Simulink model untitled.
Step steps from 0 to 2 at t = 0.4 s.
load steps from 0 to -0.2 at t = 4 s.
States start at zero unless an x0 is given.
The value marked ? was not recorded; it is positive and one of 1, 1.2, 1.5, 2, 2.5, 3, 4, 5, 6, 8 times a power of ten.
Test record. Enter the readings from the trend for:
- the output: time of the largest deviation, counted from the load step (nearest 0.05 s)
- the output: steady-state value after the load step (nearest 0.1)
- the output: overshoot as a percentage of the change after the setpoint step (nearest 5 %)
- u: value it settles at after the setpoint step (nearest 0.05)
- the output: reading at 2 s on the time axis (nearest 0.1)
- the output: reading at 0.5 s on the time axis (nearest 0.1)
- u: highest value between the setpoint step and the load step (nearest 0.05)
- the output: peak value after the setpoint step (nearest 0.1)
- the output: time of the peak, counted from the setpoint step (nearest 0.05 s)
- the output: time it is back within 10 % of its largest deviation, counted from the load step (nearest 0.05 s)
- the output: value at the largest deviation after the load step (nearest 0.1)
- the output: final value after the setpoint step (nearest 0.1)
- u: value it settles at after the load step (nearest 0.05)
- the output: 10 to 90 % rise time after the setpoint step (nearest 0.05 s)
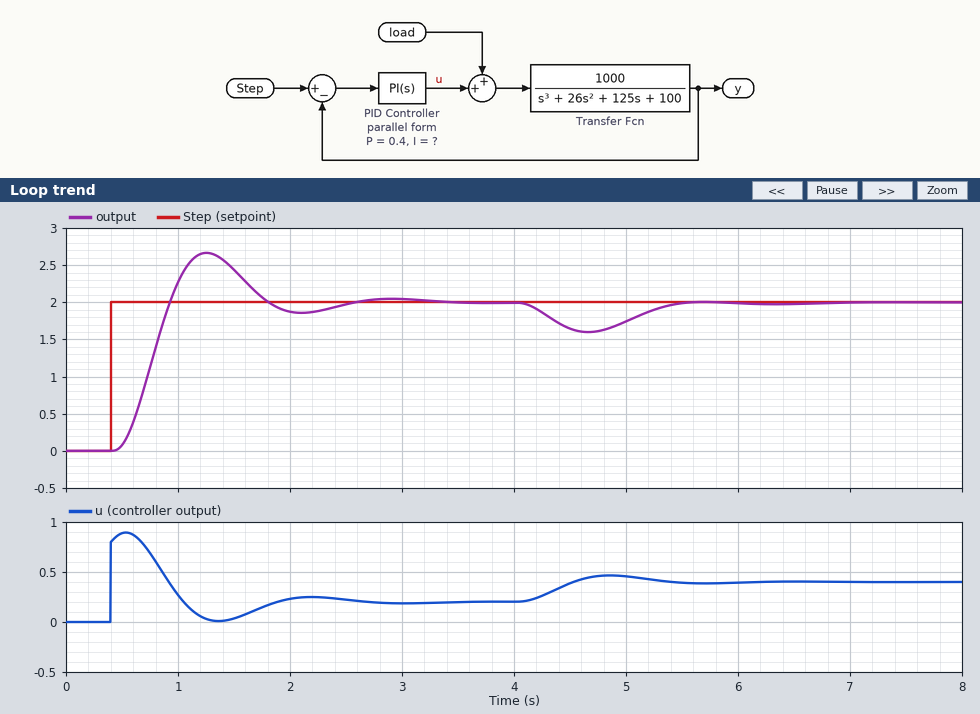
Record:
0.65 s
2.0
35 %
0.20
1.9
0.1
0.90
2.7
0.85 s
1.40 s
1.6
2.0
0.40
0.35 s
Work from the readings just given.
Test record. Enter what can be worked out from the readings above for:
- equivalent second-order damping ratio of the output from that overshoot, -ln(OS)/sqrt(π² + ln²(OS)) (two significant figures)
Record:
0.32
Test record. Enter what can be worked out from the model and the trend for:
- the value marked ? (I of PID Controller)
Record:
0.6
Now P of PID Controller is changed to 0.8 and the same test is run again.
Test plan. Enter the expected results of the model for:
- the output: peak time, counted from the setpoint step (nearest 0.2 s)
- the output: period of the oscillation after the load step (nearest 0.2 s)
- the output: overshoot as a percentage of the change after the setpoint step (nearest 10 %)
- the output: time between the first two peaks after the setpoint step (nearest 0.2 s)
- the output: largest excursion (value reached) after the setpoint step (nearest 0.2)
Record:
0.6 s
1.0 s
40 %
1.0 s
2.8
